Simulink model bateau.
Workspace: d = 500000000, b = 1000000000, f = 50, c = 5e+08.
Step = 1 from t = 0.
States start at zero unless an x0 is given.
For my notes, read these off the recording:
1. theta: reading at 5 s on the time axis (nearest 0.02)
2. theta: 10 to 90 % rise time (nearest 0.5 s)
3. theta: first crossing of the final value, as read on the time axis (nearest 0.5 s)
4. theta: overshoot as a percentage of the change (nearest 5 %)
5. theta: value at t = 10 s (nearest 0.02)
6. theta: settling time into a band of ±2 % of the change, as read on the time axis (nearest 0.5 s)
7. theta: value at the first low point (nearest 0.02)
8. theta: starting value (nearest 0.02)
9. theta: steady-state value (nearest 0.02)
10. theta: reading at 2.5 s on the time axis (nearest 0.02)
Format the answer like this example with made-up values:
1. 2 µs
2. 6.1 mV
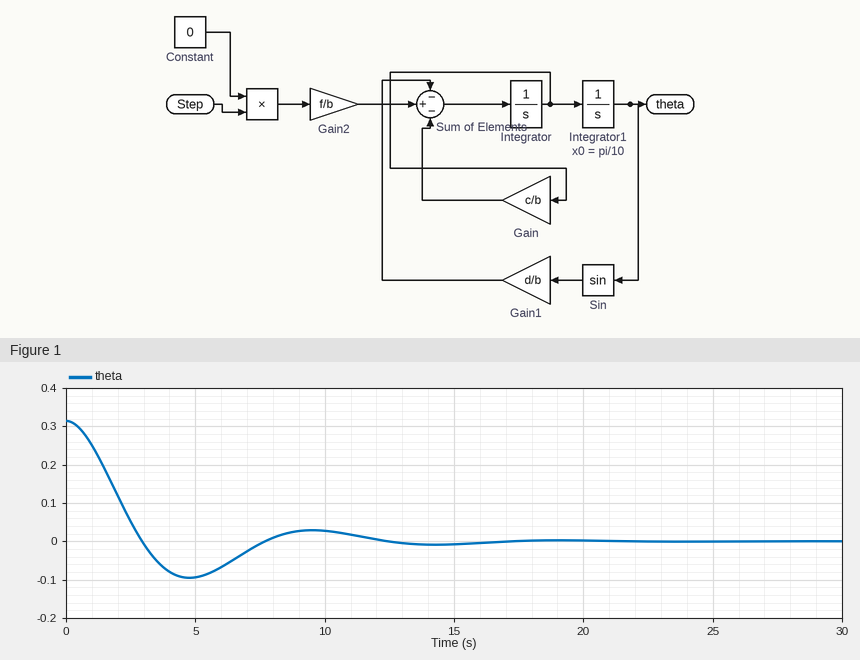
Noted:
1. -0.10
2. 2.0 s
3. 3.0 s
4. 30 %
5. 0.02
6. 15.5 s
7. -0.10
8. 0.32
9. 0.00
10. 0.06
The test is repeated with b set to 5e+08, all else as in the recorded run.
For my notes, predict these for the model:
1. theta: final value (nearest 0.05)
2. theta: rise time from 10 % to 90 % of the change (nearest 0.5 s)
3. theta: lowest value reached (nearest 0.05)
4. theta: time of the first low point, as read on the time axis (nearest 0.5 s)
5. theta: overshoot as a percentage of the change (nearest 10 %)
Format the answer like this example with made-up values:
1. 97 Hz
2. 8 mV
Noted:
1. 0.00
2. 1.5 s
3. -0.05
4. 3.5 s
5. 20 %
